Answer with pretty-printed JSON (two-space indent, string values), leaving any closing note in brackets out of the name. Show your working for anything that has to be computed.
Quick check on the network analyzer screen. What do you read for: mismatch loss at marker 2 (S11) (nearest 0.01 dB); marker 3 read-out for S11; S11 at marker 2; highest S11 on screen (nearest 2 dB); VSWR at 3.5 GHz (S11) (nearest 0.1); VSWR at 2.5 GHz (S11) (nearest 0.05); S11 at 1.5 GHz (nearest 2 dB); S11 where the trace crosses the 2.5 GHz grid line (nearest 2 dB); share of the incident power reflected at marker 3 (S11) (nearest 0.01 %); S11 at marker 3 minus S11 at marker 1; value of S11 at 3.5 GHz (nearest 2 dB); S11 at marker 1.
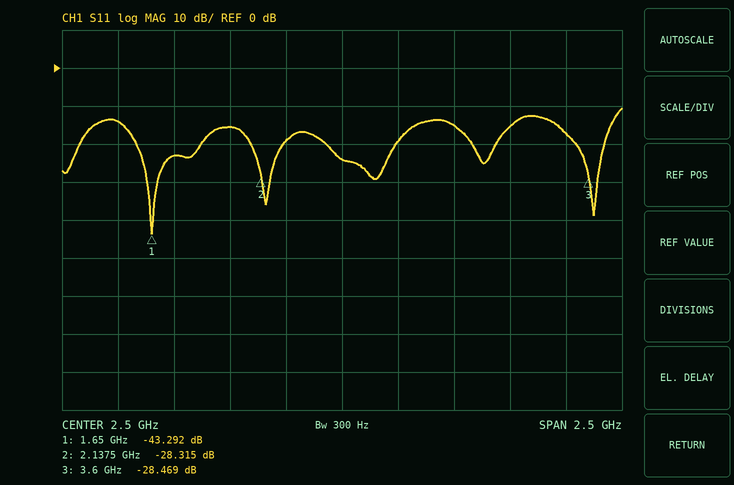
{
  "mismatch loss at marker 2 (S11)": "−10 log10(1 − 10^(-28.315/10)) ≈ 0.01 dB",
  "marker 3 read-out for S11": "-28.469 dB",
  "S11 at marker 2": "-28.315 dB",
  "highest S11 on screen": "-10 dB",
  "VSWR at 3.5 GHz (S11)": "|Γ| = 10^(-18/20) = 0.1259; VSWR = (1 + 0.1259)/(1 − 0.1259) ≈ 1.3",
  "VSWR at 2.5 GHz (S11)": "|Γ| = 10^(-24/20) = 0.0631; VSWR = (1 + 0.0631)/(1 − 0.0631) ≈ 1.13, so 1.15 to the nearest 0.05",
  "S11 at 1.5 GHz": "-14 dB",
  "S11 where the trace crosses the 2.5 GHz grid line": "-24 dB",
  "share of the incident power reflected at marker 3 (S11)": "10^(-28.469/10) ≈ 0.14 %",
  "S11 at marker 3 minus S11 at marker 1": "-28.469 − (-43.292) = 14.823 dB",
  "value of S11 at 3.5 GHz": "-18 dB",
  "S11 at marker 1": "-43.292 dB"
}
